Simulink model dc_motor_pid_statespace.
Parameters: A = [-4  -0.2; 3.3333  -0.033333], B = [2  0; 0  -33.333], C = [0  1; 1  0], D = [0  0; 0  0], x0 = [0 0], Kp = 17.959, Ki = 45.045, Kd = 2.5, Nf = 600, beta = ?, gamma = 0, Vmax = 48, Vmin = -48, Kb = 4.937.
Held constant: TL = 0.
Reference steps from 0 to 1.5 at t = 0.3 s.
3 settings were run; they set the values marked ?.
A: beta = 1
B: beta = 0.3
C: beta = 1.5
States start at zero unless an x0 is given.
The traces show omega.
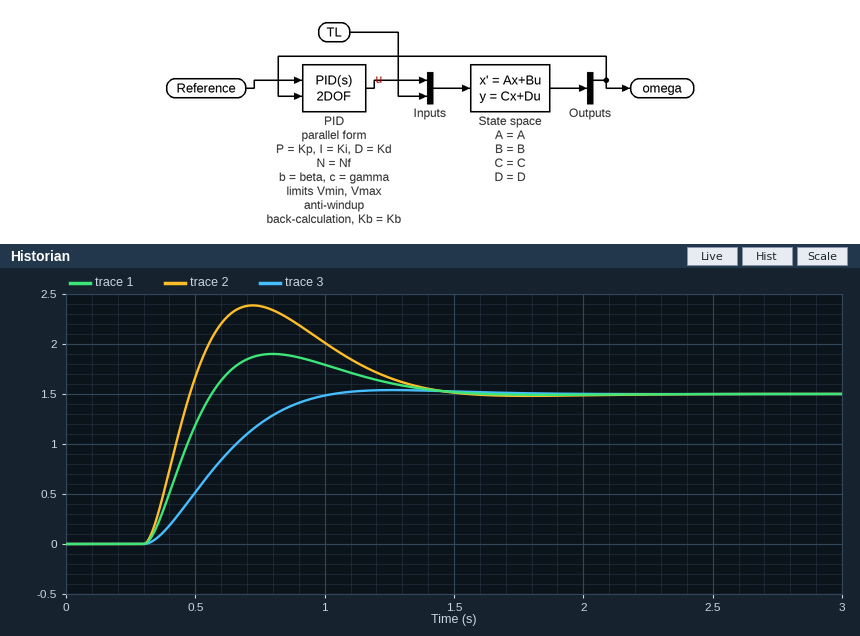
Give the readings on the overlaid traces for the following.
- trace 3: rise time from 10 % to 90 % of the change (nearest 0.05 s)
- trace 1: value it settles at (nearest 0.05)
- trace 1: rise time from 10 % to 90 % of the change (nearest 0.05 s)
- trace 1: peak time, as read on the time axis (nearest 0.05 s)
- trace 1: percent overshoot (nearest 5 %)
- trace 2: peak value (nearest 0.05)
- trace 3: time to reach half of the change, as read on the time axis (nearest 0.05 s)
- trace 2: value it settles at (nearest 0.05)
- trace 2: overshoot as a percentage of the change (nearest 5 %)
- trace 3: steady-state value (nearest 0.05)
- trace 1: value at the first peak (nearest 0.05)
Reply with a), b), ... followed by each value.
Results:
a) 0.45 s
b) 1.50
c) 0.20 s
d) 0.80 s
e) 25 %
f) 2.40
g) 0.55 s
h) 1.50
i) 60 %
j) 1.50
k) 1.90
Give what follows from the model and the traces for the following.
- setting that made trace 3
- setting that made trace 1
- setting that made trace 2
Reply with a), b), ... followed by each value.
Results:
a) B
b) A
c) C
